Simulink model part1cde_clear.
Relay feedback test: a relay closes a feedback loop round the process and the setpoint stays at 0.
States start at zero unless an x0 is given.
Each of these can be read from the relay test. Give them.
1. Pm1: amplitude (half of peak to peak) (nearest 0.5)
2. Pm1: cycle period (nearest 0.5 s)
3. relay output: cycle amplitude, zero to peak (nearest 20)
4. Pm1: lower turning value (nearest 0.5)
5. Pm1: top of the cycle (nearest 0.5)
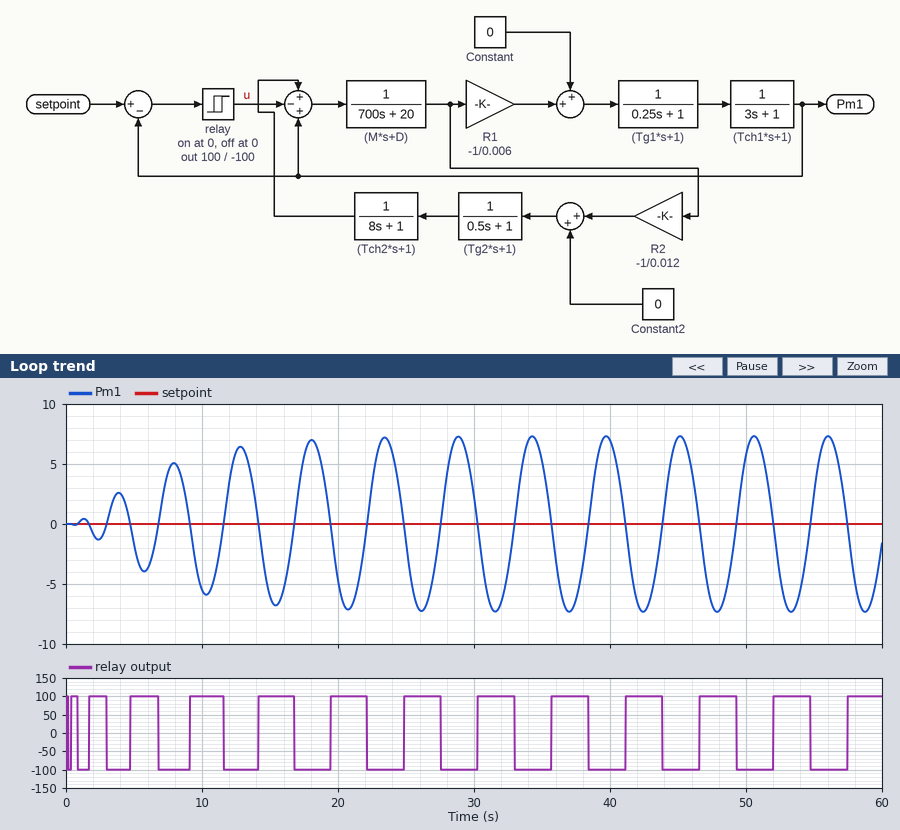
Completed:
7.5
5.5 s
100
-7.5
7.5
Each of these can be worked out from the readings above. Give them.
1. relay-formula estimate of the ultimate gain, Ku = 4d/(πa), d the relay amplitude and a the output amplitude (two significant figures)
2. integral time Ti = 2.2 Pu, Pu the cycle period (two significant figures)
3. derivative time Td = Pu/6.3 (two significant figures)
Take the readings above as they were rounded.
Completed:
17
12 s
0.87 s
